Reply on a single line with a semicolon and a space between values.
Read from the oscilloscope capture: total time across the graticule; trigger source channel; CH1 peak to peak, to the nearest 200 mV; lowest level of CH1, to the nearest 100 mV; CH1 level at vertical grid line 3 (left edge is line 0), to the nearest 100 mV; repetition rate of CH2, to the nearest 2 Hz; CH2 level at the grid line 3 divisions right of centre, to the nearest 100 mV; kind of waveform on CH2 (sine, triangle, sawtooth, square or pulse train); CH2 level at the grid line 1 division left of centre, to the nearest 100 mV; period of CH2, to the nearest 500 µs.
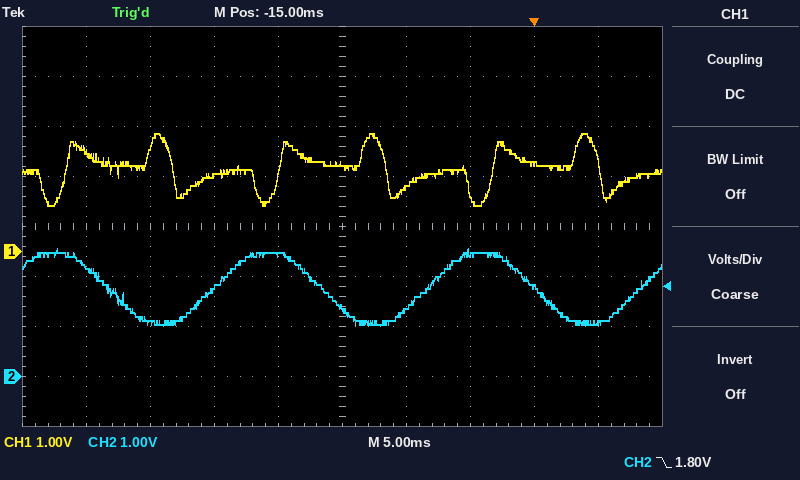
50 ms; CH2; 1.4 V; 900 mV; 1.5 V; 60 Hz; 1.8 V; sine; 2.4 V; 16.5 ms
